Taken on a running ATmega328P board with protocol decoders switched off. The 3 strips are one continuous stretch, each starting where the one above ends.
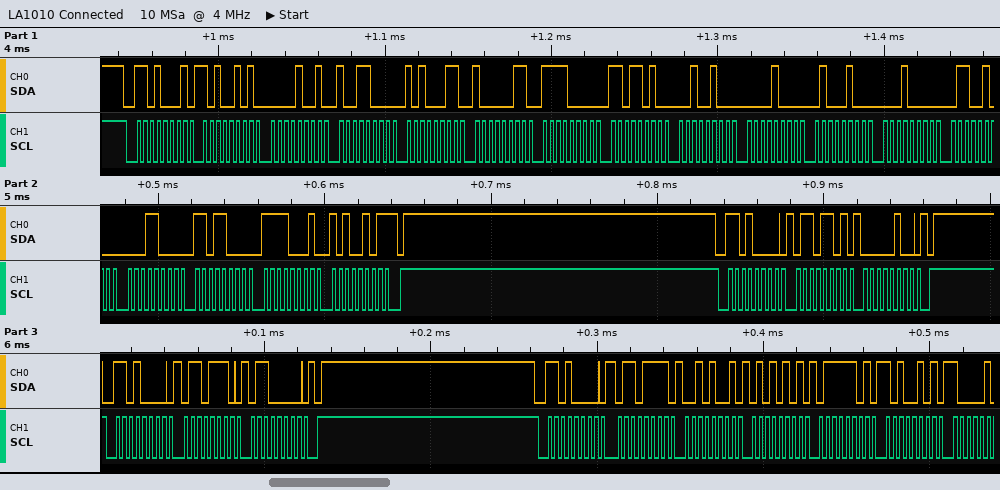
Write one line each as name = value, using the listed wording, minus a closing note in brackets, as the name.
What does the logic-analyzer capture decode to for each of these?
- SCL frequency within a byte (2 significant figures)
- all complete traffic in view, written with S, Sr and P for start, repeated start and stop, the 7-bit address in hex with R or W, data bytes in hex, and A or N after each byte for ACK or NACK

SCL frequency within a byte = 250 kHz
all complete traffic in view, written with S, Sr and P for start, repeated start and stop, the 7-bit address in hex with R or W, data bytes in hex, and A or N after each byte for ACK or NACK = S 68R A A5 A 09 A 98 A A3 A 83 A F0 A DA A 24 A 08 A 44 A 10 A 64 A 18 A D8 A F1 A A5 N P S 68W A 6D A 04 A P S 68W A 6E A 60 A P S 68W A 6F A 29 A 55 A 7D A A5 A
